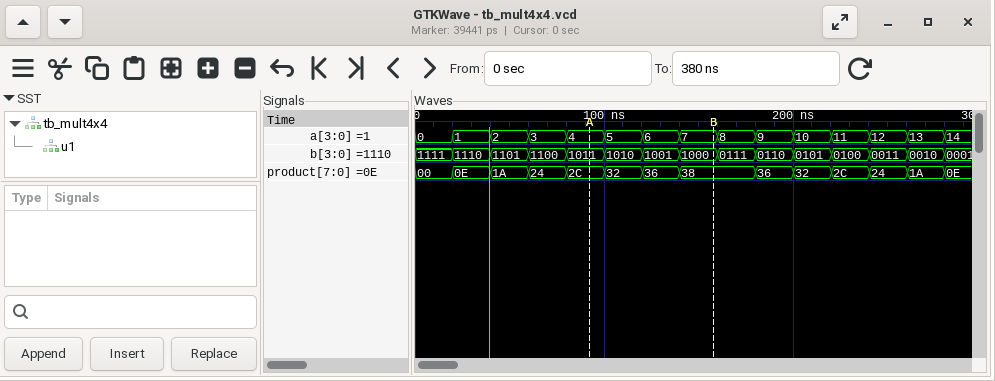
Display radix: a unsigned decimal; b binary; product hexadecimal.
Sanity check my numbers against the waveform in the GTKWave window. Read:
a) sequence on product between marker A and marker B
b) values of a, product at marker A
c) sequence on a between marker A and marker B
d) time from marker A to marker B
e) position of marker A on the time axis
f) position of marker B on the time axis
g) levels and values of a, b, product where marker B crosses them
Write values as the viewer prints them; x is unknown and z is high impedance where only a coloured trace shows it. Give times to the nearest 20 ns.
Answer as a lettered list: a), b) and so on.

a) 2C, 32, 36, 38
b) a=4, product=2C
c) 4, 5, 6, 7
d) 60 ns
e) 100 ns
f) 160 ns
g) a=7, b=1000, product=38
